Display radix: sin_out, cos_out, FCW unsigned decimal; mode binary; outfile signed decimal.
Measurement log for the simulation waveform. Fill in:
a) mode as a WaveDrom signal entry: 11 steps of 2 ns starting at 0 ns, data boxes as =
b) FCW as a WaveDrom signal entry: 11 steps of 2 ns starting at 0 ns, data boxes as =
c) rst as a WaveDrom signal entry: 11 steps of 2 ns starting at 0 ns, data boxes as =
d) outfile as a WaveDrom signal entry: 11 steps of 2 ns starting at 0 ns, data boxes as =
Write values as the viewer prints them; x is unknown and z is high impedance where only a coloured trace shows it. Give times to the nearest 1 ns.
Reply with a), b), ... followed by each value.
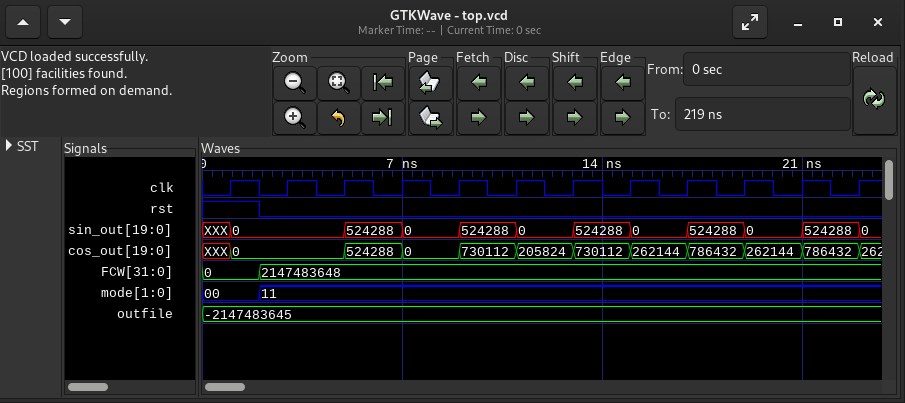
a) {name: 'mode', wave: '==.........', data: '00 11'}
b) {name: 'FCW', wave: '==.........', data: '0 2147483648'}
c) {name: 'rst', wave: '10.........'}
d) {name: 'outfile', wave: '=..........', data: '-2147483645'}
